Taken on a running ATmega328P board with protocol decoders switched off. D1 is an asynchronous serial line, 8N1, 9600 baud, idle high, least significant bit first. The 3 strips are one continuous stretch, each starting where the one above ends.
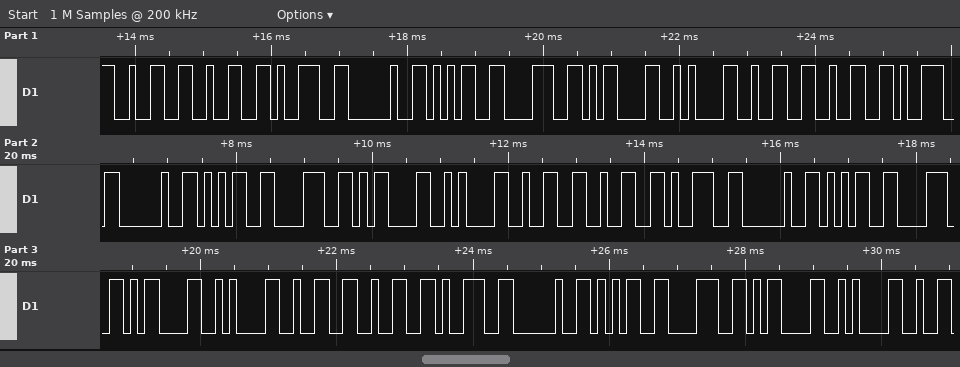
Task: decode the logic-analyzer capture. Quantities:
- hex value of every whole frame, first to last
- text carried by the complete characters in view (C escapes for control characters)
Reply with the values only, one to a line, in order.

32 32 39 20 35 38 0D 0A 32 32 39 20 35 38 0D 0A 32 32 39 20 35 38 0D 0A 32 32 39 20 35 38 0D 0A
"229 58\r\n229 58\r\n229 58\r\n229 58\r\n"
